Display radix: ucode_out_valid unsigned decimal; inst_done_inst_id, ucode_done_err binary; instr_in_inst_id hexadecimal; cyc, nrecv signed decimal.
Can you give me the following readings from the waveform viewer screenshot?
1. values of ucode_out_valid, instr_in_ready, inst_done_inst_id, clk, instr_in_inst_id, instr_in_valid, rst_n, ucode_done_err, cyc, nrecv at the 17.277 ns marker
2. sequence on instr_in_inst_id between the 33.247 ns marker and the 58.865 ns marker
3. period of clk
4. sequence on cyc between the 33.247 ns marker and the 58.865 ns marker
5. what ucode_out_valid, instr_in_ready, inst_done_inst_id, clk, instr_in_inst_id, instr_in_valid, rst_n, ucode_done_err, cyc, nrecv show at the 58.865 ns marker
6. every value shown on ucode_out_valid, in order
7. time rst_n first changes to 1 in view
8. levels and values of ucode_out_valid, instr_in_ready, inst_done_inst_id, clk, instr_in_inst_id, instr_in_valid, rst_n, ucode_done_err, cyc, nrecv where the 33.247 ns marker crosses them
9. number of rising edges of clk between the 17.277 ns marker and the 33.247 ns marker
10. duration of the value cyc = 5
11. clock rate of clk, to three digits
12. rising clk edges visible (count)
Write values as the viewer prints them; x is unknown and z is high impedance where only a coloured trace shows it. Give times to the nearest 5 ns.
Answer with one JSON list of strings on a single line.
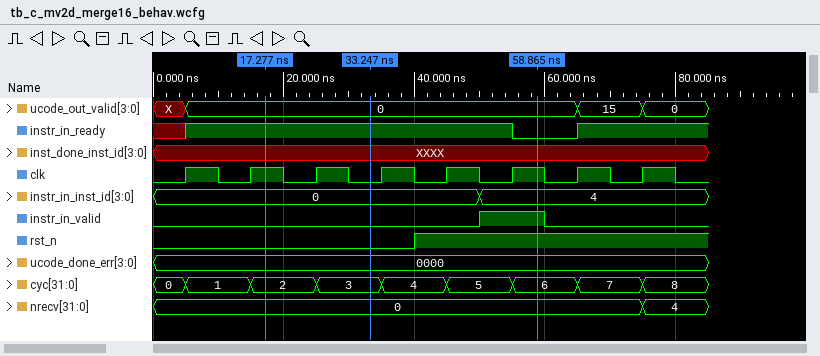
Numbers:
["ucode_out_valid=0, instr_in_ready=1, inst_done_inst_id=XXXX, clk=1, instr_in_inst_id=0, instr_in_valid=0, rst_n=0, ucode_done_err=0000, cyc=2, nrecv=0", "0, 4", "10 ns", "3, 4, 5, 6", "ucode_out_valid=0, instr_in_ready=0, inst_done_inst_id=XXXX, clk=1, instr_in_inst_id=4, instr_in_valid=1, rst_n=1, ucode_done_err=0000, cyc=6, nrecv=0", "X, 0, 15, 0", "40 ns", "ucode_out_valid=0, instr_in_ready=1, inst_done_inst_id=XXXX, clk=0, instr_in_inst_id=0, instr_in_valid=0, rst_n=0, ucode_done_err=0000, cyc=3, nrecv=0", "1", "10 ns", "100 MHz", "8"]
